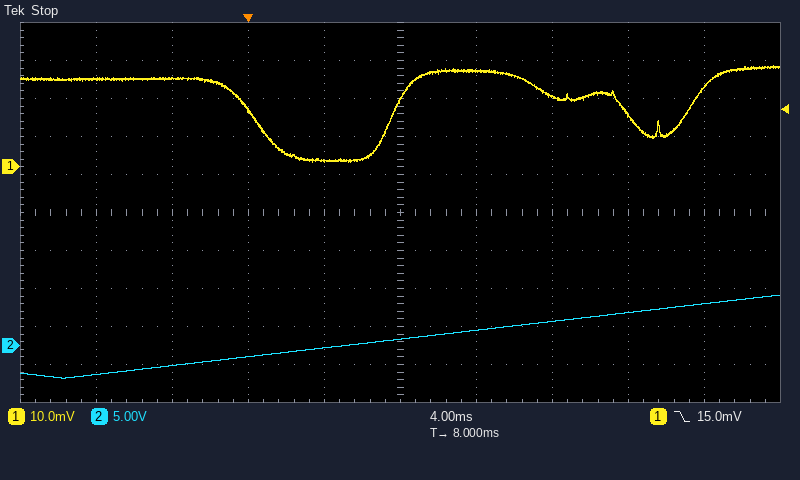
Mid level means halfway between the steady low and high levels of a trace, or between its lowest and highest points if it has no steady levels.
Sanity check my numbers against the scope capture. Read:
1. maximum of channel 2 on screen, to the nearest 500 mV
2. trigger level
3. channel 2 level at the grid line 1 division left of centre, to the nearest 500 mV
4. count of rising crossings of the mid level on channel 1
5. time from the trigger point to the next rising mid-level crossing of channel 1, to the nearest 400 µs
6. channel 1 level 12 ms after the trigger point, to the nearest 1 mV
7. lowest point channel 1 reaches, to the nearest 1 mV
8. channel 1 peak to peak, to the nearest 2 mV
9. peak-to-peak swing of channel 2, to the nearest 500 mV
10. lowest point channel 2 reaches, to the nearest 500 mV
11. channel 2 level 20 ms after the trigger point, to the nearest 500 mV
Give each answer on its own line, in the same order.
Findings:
6.5 V
15.0 mV
-500 mV
2
7.6 ms
25 mV
1 mV
26 mV
11.0 V
-4.5 V
4.5 V
